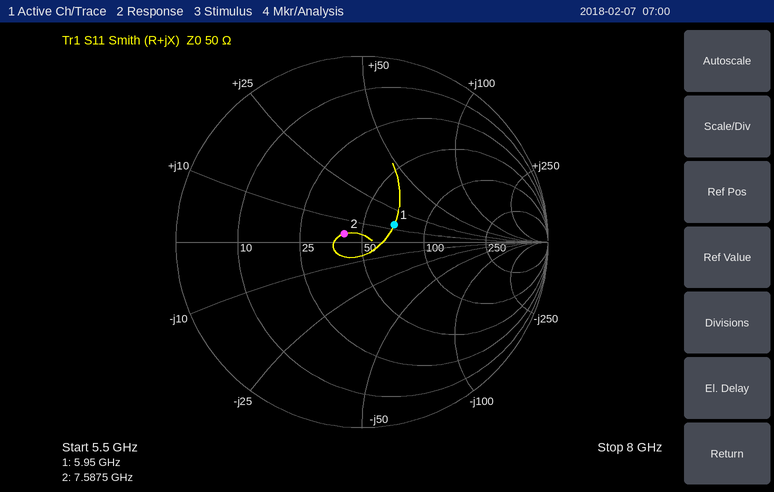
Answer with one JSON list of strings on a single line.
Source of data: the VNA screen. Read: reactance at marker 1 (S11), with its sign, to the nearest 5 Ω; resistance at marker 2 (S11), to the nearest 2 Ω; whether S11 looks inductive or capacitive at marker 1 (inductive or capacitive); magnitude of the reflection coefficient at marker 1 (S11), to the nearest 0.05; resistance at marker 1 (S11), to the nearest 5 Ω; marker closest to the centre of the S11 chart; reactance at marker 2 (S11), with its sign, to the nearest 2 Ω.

["+15 Ω", "42 Ω", "inductive", "0.20", "70 Ω", "marker 2", "+4 Ω"]
